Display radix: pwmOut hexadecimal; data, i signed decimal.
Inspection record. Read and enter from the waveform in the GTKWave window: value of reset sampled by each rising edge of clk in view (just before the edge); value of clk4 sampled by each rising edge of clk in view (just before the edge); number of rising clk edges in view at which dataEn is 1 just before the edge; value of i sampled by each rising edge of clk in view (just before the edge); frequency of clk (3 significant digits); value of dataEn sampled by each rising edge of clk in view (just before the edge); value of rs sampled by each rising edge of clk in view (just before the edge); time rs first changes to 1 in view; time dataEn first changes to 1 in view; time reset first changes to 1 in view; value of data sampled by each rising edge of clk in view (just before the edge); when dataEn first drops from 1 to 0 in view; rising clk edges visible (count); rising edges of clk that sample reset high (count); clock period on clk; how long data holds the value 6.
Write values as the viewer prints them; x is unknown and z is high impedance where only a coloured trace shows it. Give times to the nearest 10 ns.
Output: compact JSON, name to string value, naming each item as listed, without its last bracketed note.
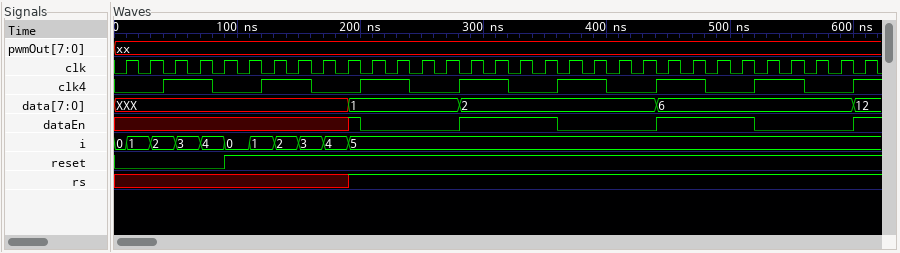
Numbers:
{"value of reset sampled by each rising edge of clk in view": "0 0 0 0 0 1 1 1 1 1 1 1 1 1 1 1 1 1 1 1 1 1 1 1 1 1 1 1 1 1 1", "value of clk4 sampled by each rising edge of clk in view": "0 0 1 1 0 0 1 1 0 0 1 1 0 0 1 1 0 0 1 1 0 0 1 1 0 0 1 1 0 0 1", "number of rising clk edges in view at which dataEn is 1 just before the edge": "9", "value of i sampled by each rising edge of clk in view": "0, 1, 2, 3, 4, 0, 1, 2, 3, 4, 5, 5, 5, 5, 5, 5, 5, 5, 5, 5, 5, 5, 5, 5, 5, 5, 5, 5, 5, 5, 5", "frequency of clk": "50.0 MHz", "value of dataEn sampled by each rising edge of clk in view": "x x x x x x x x x x 0 0 0 0 1 1 1 1 0 0 0 0 1 1 1 1 0 0 0 0 1", "value of rs sampled by each rising edge of clk in view": "x x x x x x x x x x 1 1 1 1 1 1 1 1 1 1 1 1 1 1 1 1 1 1 1 1 1", "time rs first changes to 1 in view": "190 ns", "time dataEn first changes to 1 in view": "190 ns", "time reset first changes to 1 in view": "90 ns", "value of data sampled by each rising edge of clk in view": "XXX, XXX, XXX, XXX, XXX, XXX, XXX, XXX, XXX, XXX, 1, 1, 1, 1, 2, 2, 2, 2, 2, 2, 2, 2, 6, 6, 6, 6, 6, 6, 6, 6, 12", "when dataEn first drops from 1 to 0 in view": "200 ns", "rising clk edges visible": "31", "rising edges of clk that sample reset high": "26", "clock period on clk": "20 ns", "how long data holds the value 6": "160 ns"}
